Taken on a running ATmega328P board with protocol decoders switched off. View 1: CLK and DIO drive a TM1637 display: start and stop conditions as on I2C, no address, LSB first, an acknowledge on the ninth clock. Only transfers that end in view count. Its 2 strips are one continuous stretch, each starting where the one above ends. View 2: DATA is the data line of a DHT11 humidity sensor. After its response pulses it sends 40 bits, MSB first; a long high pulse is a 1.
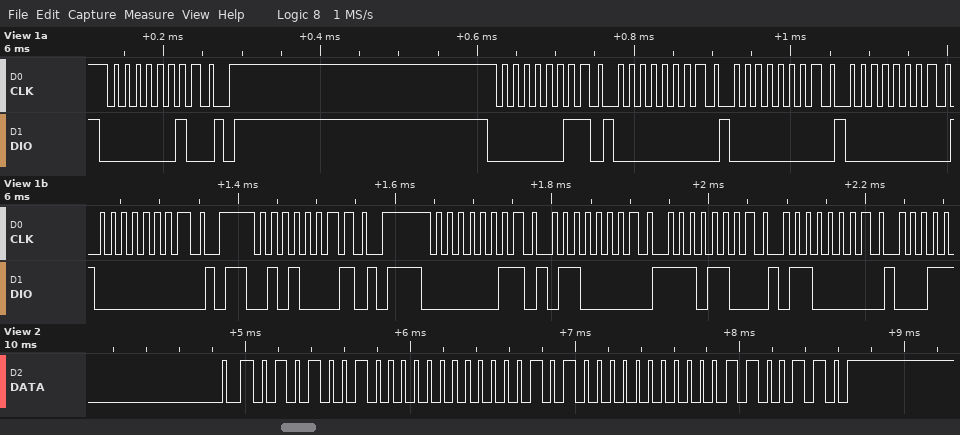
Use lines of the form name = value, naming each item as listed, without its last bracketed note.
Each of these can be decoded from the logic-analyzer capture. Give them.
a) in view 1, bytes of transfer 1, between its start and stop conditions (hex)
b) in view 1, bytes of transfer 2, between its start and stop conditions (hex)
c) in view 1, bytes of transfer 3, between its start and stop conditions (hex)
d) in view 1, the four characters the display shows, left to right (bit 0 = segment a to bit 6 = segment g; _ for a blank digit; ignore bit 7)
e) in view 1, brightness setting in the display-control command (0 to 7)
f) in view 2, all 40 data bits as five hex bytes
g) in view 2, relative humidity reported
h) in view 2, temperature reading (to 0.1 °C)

in view 1, bytes of transfer 1, between its start and stop conditions = 40
in view 1, bytes of transfer 2, between its start and stop conditions = C0 00 00 00 00
in view 1, bytes of transfer 3, between its start and stop conditions = 8A
in view 1, the four characters the display shows, left to right = ____
in view 1, brightness setting in the display-control command = 2
in view 2, all 40 data bits as five hex bytes = 52 00 14 00 66
in view 2, relative humidity reported = 82 %
in view 2, temperature reading = 20.0 °C
